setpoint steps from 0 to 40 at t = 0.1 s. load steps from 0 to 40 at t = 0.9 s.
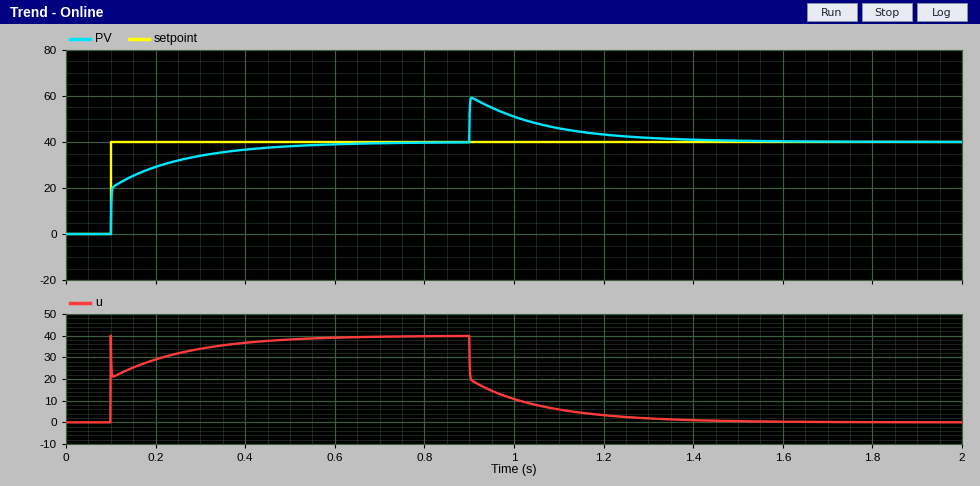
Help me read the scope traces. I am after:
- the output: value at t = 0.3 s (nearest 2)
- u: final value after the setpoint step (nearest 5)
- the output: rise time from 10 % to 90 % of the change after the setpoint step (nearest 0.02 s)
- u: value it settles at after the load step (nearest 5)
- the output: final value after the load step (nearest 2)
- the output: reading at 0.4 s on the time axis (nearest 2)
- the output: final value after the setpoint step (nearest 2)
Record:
34
40
0.26 s
0
40
36
40
